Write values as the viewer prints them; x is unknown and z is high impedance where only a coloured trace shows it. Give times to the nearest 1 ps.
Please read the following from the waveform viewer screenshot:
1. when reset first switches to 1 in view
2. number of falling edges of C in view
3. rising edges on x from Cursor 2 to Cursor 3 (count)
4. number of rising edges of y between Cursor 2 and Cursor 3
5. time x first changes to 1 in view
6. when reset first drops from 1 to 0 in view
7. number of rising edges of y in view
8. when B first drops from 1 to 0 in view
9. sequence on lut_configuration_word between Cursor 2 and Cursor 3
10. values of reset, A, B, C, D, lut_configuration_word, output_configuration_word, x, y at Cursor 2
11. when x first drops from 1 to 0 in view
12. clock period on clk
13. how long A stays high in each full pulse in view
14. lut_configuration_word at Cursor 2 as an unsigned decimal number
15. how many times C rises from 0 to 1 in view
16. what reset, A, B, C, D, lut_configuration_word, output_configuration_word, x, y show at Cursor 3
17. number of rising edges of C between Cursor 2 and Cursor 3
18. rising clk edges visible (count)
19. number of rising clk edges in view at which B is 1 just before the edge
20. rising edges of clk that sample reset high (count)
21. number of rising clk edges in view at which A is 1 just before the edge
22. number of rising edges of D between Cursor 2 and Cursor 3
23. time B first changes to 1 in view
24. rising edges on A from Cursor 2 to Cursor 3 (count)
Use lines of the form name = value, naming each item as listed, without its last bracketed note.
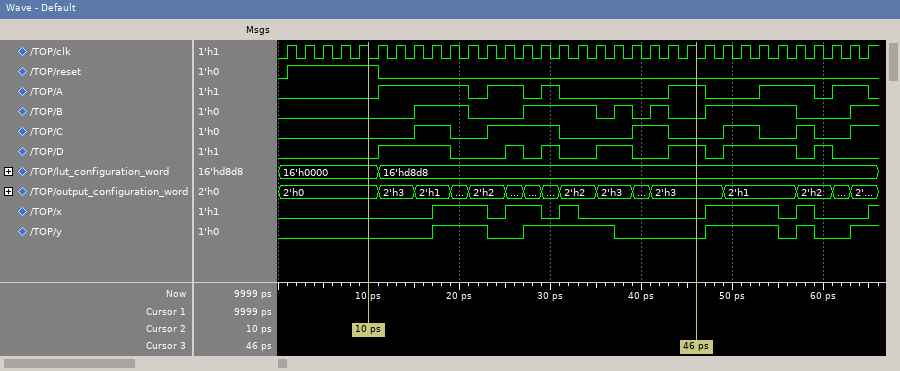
when reset first switches to 1 in view = 1 ps
number of falling edges of C in view = 5
rising edges on x from Cursor 2 to Cursor 3 = 3
number of rising edges of y between Cursor 2 and Cursor 3 = 2
time x first changes to 1 in view = 17 ps
when reset first drops from 1 to 0 in view = 11 ps
number of rising edges of y in view = 5
when B first drops from 1 to 0 in view = 21 ps
sequence on lut_configuration_word between Cursor 2 and Cursor 3 = 16'h0000, 16'hd8d8
values of reset, A, B, C, D, lut_configuration_word, output_configuration_word, x, y at Cursor 2 = reset=1, A=0, B=0, C=0, D=0, lut_configuration_word=16'h0000, output_configuration_word=2'h0, x=0, y=0
when x first drops from 1 to 0 in view = 23 ps
clock period on clk = 2 ps
how long A stays high in each full pulse in view = 10 ps, 4 ps, 2 ps, 4 ps, 6 ps, 4 ps
lut_configuration_word at Cursor 2 as an unsigned decimal number = 0
how many times C rises from 0 to 1 in view = 6
what reset, A, B, C, D, lut_configuration_word, output_configuration_word, x, y show at Cursor 3 = reset=0, A=1, B=0, C=0, D=1, lut_configuration_word=16'hd8d8, output_configuration_word=2'h3, x=0, y=0
number of rising edges of C between Cursor 2 and Cursor 3 = 3
rising clk edges visible = 33
number of rising clk edges in view at which B is 1 just before the edge = 15
rising edges of clk that sample reset high = 5
number of rising clk edges in view at which A is 1 just before the edge = 15
number of rising edges of D between Cursor 2 and Cursor 3 = 5
time B first changes to 1 in view = 15 ps
rising edges on A from Cursor 2 to Cursor 3 = 4
